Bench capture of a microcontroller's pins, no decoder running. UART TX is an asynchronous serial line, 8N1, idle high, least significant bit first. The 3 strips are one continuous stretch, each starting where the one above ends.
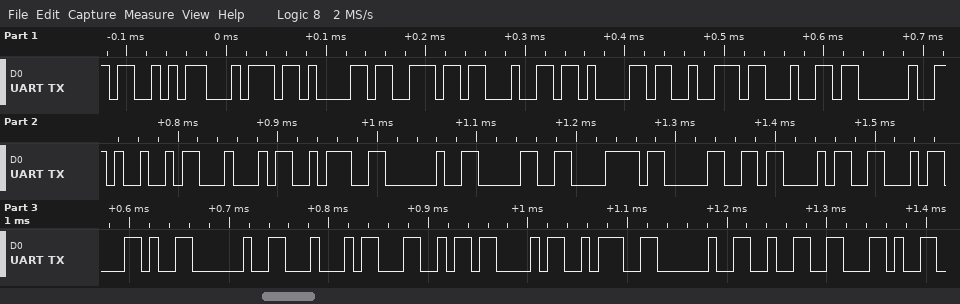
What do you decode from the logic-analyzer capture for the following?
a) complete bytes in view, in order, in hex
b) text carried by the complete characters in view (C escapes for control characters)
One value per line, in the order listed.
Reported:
53 74 61 6E 64 61 72 64 20 49 44 3A 20 30 78 30 43 46 2C 20 44 4C 43 3A 20 32 2C
"Standard ID: 0x0CF, DLC: 2,"
